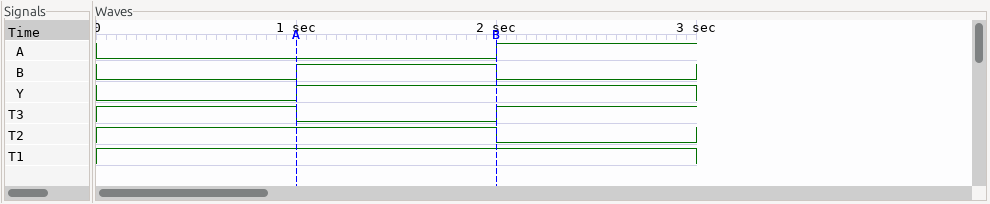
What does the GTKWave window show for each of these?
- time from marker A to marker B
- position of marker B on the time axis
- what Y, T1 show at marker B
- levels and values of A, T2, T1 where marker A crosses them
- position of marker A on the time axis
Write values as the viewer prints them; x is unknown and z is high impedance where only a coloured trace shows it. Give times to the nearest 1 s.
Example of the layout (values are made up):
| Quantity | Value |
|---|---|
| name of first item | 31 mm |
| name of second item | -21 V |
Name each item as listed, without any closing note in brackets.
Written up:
| Quantity | Value |
|---|---|
| time from marker A to marker B | 1 s |
| position of marker B on the time axis | 2 s |
| what Y, T1 show at marker B | Y=1, T1=1 |
| levels and values of A, T2, T1 where marker A crosses them | A=0, T2=1, T1=1 |
| position of marker A on the time axis | 1 s |
